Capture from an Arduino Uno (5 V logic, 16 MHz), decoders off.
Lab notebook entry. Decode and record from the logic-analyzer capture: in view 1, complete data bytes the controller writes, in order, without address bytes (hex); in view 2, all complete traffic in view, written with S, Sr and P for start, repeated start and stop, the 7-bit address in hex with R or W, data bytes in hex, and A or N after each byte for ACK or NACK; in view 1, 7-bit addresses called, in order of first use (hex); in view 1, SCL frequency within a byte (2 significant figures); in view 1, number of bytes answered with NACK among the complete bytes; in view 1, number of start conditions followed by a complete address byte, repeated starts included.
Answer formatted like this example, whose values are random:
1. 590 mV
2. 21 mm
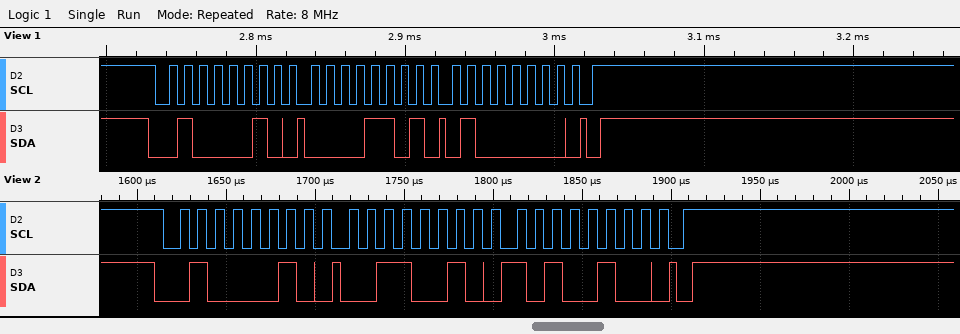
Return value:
1. 0D 40
2. S 21W A 32 A A4 A P
3. 0x21
4. 100 kHz
5. 0
6. 1
